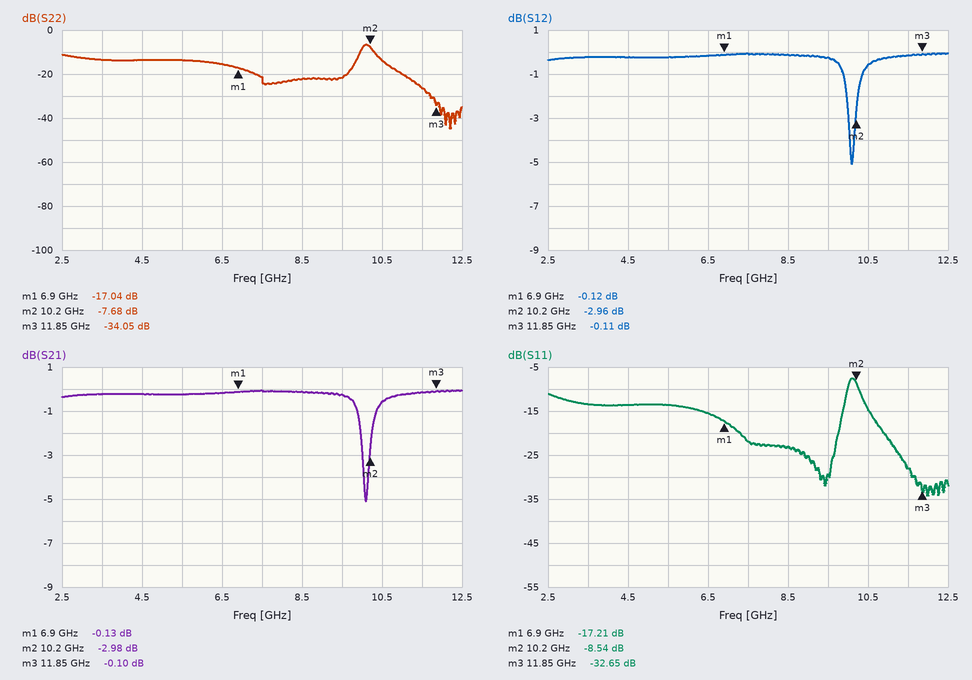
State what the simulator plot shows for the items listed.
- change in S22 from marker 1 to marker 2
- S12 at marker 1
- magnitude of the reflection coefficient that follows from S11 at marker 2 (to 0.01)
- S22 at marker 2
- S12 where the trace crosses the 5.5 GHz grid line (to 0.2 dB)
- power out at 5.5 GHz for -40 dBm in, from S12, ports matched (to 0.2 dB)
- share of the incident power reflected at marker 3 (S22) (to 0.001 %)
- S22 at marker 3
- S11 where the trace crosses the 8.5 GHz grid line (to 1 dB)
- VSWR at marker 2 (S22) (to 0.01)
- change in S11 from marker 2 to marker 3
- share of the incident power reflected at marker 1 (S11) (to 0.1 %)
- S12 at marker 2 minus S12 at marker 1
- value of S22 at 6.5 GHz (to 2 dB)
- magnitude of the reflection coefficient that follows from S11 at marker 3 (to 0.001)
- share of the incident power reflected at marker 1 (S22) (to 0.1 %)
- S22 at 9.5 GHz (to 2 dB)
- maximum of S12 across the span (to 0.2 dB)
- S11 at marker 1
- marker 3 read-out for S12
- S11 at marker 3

9.36 dB
-0.12 dB
0.37
-7.68 dB
-0.2 dB
-40.2 dBm
0.039 %
-34.05 dB
-23 dB
2.41
-24.11 dB
1.9 %
-2.84 dB
-16 dB
0.023
2.0 %
-22 dB
0.0 dB
-17.21 dB
-0.11 dB
-32.65 dB
